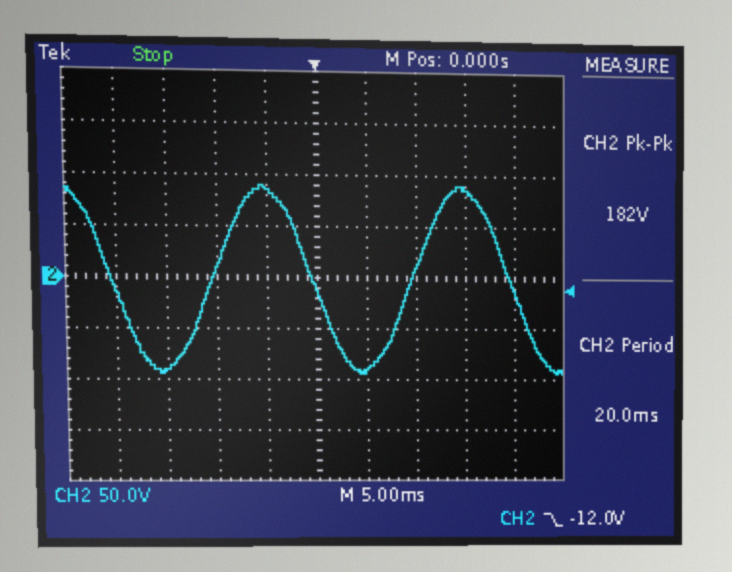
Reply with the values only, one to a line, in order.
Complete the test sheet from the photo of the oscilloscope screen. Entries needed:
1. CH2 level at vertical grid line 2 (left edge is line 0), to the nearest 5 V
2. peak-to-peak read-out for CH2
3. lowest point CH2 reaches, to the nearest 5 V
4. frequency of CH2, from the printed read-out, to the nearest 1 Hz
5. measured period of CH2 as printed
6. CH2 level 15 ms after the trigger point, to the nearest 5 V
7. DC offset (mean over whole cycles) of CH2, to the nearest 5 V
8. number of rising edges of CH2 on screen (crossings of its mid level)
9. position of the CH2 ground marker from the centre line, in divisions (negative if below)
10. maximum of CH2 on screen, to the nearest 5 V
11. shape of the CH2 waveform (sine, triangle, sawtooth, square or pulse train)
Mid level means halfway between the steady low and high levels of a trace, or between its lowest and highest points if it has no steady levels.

-90 V
182 V
-95 V
50 Hz
20.0 ms
85 V
0 V
2
0.0 div
90 V
sine
